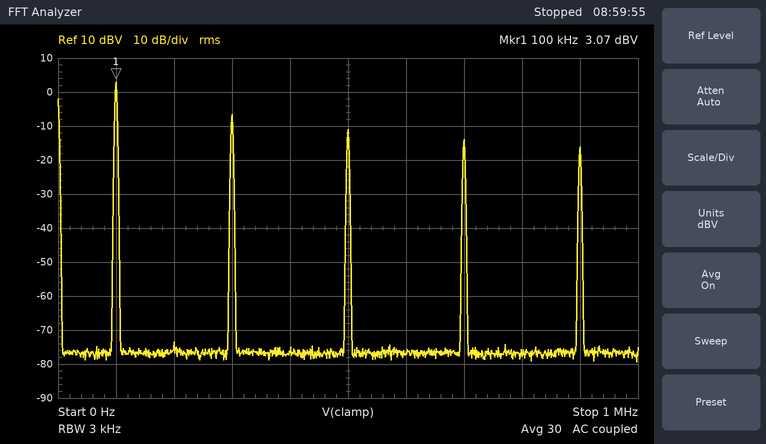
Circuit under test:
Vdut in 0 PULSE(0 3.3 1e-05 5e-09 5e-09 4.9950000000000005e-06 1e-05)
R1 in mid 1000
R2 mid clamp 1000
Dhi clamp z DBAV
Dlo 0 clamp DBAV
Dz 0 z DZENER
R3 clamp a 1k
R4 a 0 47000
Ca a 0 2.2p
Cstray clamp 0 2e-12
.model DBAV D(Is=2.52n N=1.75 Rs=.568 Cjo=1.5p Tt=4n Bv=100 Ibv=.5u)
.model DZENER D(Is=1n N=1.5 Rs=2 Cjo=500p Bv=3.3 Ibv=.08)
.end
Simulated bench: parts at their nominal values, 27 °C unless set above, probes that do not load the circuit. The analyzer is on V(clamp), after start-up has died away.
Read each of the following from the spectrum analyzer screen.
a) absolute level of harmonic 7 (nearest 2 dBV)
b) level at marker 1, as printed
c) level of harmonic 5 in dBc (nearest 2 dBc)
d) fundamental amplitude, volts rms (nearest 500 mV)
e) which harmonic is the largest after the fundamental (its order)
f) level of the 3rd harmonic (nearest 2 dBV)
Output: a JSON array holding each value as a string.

["-14 dBV", "3.07 dBV", "-14 dBc", "1.5 V", "3", "-6 dBV"]
